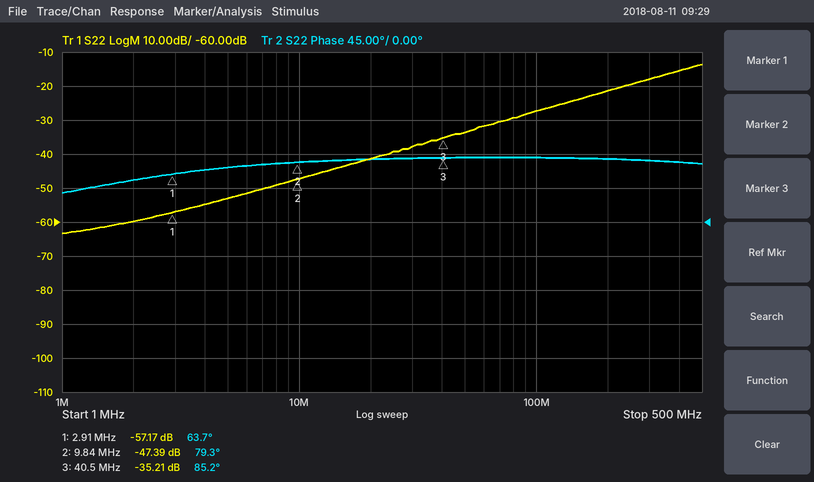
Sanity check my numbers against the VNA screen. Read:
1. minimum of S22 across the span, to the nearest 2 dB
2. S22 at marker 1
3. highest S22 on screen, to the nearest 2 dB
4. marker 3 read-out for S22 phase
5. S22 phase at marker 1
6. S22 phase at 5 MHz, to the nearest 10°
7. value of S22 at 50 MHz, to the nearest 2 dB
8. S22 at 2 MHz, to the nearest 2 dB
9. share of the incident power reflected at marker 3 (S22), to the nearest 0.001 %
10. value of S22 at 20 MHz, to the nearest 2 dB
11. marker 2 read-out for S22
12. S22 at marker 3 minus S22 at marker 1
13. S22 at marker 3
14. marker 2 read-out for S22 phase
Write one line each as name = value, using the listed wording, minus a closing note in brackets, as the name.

minimum of S22 across the span, to the nearest 2 dB = -64 dB
S22 at marker 1 = -57.17 dB
highest S22 on screen, to the nearest 2 dB = -14 dB
marker 3 read-out for S22 phase = 85.2°
S22 phase at marker 1 = 63.7°
S22 phase at 5 MHz, to the nearest 10° = 70°
value of S22 at 50 MHz, to the nearest 2 dB = -34 dB
S22 at 2 MHz, to the nearest 2 dB = -60 dB
share of the incident power reflected at marker 3 (S22), to the nearest 0.001 % = 0.030 %
value of S22 at 20 MHz, to the nearest 2 dB = -42 dB
marker 2 read-out for S22 = -47.39 dB
S22 at marker 3 minus S22 at marker 1 = 21.96 dB
S22 at marker 3 = -35.21 dB
marker 2 read-out for S22 phase = 79.3°
